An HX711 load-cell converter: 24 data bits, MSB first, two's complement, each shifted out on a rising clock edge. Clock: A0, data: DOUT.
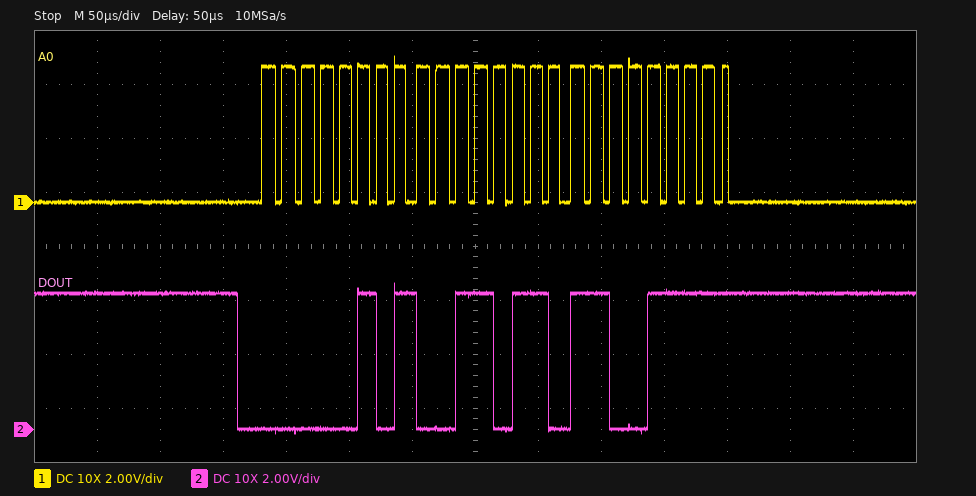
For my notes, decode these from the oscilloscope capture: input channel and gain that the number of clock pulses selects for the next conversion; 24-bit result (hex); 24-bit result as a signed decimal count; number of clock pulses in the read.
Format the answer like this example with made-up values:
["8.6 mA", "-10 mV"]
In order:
["channel A, gain 128", "0x0536CF", "341711", "25"]
